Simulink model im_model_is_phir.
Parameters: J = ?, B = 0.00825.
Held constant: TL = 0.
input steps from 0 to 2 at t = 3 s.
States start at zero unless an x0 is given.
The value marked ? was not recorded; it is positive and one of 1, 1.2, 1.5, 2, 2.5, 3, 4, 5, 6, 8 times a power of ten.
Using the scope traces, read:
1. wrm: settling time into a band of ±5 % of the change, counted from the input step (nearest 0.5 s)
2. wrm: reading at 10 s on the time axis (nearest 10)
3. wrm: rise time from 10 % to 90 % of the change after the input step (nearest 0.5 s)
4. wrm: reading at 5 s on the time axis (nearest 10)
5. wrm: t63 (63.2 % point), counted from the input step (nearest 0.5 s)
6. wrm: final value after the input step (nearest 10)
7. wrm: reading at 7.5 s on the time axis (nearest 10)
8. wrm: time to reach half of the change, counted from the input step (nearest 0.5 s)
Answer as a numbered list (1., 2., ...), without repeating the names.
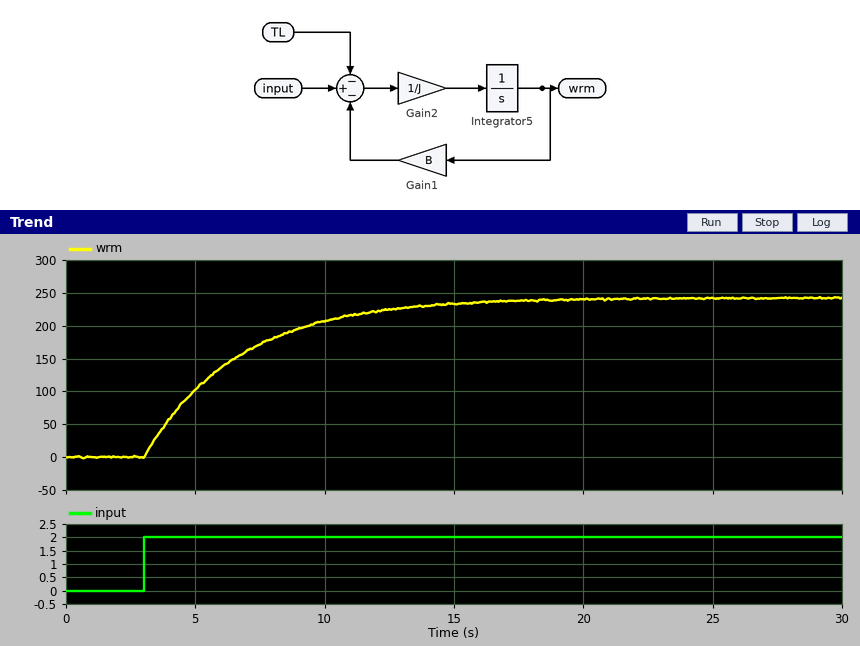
1. 11.0 s
2. 210
3. 8.0 s
4. 100
5. 3.5 s
6. 240
7. 170
8. 2.5 s
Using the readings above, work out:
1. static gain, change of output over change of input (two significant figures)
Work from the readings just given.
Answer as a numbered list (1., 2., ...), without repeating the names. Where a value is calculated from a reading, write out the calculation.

1. (240 - 0) / (2 - 0) = 120
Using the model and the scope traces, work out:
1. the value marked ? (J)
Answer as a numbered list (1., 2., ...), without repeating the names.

1. 0.03
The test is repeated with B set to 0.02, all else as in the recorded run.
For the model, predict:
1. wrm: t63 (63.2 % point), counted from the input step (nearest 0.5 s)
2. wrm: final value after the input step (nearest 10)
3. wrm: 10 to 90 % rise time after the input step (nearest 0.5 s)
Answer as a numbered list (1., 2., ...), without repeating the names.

1. 1.5 s
2. 100
3. 3.5 s
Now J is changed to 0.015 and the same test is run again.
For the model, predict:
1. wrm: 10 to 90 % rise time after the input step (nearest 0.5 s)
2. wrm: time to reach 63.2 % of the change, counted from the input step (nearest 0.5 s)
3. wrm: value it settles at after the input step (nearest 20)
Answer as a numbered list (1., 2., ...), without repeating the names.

1. 4.0 s
2. 2.0 s
3. 240
